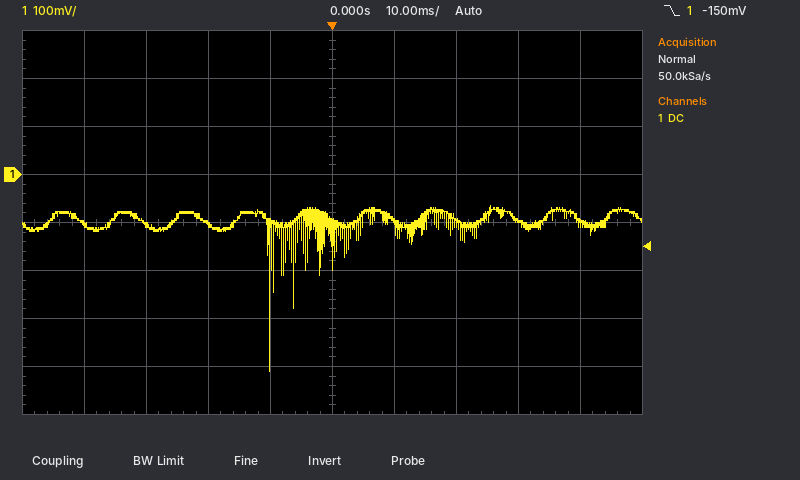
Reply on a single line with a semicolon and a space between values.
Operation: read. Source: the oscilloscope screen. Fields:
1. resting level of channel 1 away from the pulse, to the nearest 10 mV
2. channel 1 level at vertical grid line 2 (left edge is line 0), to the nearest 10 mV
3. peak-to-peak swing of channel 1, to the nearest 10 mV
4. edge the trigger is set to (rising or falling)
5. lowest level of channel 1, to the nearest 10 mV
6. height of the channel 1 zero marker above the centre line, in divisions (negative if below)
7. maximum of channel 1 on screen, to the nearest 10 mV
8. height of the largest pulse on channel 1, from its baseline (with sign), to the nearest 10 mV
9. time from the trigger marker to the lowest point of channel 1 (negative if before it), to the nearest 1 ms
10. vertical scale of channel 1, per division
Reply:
-100 mV; -100 mV; 350 mV; falling; -410 mV; +1.0 div; -60 mV; -310 mV; -10 ms; 100 mV
